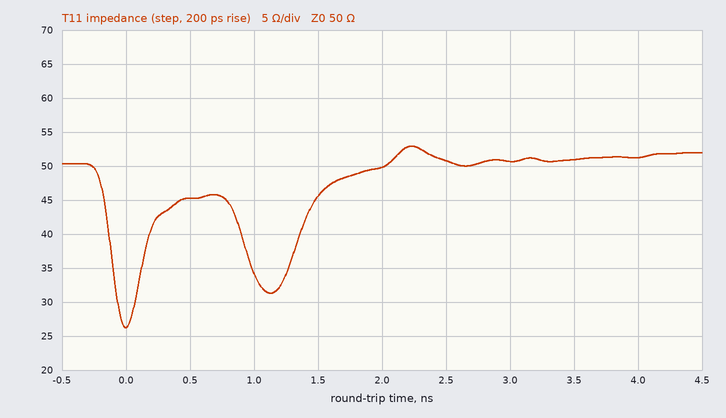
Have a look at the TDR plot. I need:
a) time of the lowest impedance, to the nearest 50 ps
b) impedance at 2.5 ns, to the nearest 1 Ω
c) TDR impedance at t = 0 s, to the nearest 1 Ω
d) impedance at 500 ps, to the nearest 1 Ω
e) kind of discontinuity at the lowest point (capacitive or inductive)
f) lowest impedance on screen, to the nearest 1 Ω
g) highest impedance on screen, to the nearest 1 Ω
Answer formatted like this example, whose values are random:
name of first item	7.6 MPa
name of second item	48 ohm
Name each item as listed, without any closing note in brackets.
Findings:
time of the lowest impedance, to the nearest 50 ps	0 ps
impedance at 2.5 ns, to the nearest 1 Ω	51 Ω
TDR impedance at t = 0 s, to the nearest 1 Ω	26 Ω
impedance at 500 ps, to the nearest 1 Ω	45 Ω
kind of discontinuity at the lowest point	capacitive
lowest impedance on screen, to the nearest 1 Ω	26 Ω
highest impedance on screen, to the nearest 1 Ω	53 Ω
